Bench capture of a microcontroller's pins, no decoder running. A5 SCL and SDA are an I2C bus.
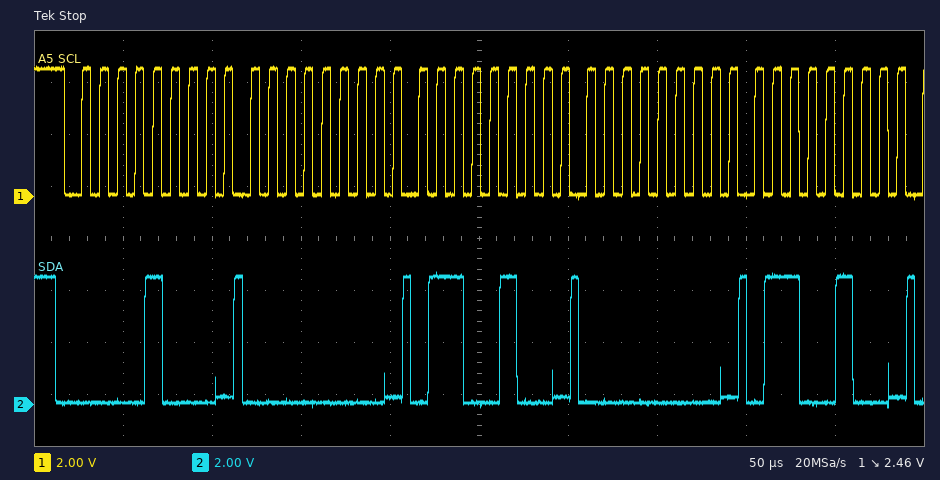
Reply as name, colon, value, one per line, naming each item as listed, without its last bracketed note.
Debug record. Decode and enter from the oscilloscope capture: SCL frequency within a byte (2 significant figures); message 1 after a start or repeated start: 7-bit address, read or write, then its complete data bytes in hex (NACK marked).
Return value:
SCL frequency within a byte: 100 kHz
message 1 after a start or repeated start: 7-bit address, read or write, then its complete data bytes in hex: 0x04 write: 00 64 00 64
